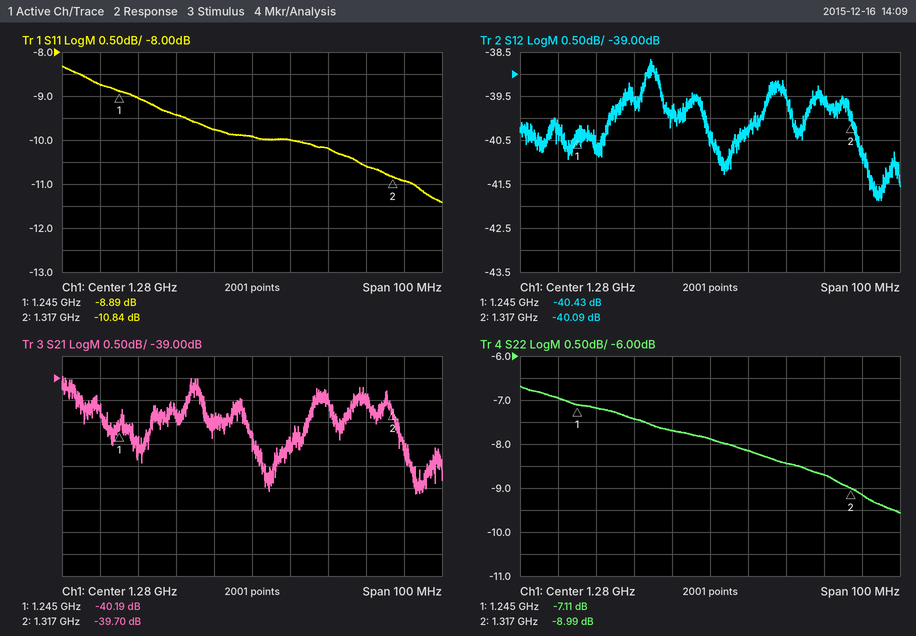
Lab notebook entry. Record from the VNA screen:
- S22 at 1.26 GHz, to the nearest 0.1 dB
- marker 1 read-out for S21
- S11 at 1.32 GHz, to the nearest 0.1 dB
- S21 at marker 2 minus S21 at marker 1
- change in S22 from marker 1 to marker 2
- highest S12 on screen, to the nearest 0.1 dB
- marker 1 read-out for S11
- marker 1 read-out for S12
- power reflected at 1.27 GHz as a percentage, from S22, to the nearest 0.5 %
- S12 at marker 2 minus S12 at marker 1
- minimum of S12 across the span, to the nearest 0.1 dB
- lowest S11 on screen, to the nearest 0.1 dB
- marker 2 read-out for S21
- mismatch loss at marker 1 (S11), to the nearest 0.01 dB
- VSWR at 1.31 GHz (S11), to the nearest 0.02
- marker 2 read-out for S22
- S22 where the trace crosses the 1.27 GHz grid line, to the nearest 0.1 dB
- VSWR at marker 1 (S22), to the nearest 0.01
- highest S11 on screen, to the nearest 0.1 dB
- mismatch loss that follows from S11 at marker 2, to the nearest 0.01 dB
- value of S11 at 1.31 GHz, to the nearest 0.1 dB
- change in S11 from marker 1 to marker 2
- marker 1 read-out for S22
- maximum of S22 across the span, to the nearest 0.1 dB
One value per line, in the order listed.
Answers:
-7.4 dB
-40.19 dB
-10.9 dB
0.49 dB
-1.88 dB
-38.7 dB
-8.89 dB
-40.43 dB
17.0 %
0.34 dB
-41.9 dB
-11.4 dB
-39.70 dB
0.60 dB
1.84
-8.99 dB
-7.7 dB
2.58
-8.3 dB
0.37 dB
-10.6 dB
-1.95 dB
-7.11 dB
-6.7 dB
